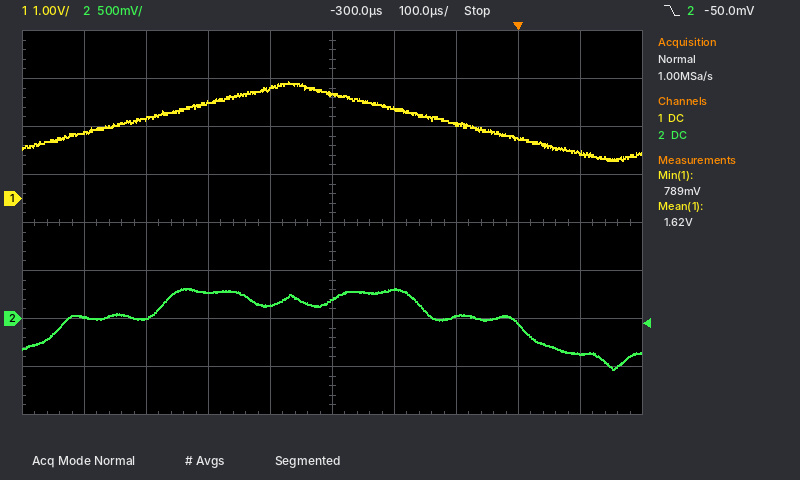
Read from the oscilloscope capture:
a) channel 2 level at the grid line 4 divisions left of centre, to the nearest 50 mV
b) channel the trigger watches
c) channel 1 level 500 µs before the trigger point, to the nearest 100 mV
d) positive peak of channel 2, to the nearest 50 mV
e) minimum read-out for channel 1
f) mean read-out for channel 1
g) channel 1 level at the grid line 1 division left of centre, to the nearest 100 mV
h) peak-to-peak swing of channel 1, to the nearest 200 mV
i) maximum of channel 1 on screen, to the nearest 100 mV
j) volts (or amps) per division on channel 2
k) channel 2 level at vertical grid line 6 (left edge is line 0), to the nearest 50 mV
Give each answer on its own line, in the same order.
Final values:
0 mV
channel 2
2.0 V
300 mV
789 mV
1.62 V
2.3 V
1.6 V
2.4 V
500 mV
300 mV
